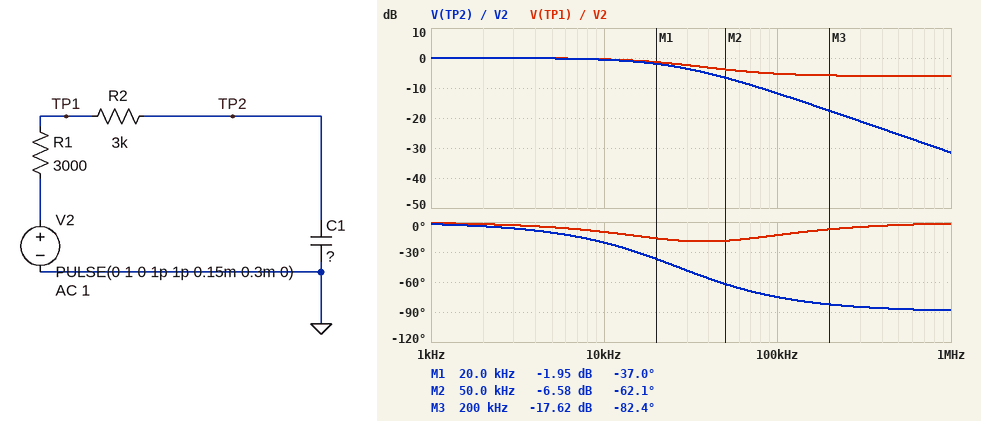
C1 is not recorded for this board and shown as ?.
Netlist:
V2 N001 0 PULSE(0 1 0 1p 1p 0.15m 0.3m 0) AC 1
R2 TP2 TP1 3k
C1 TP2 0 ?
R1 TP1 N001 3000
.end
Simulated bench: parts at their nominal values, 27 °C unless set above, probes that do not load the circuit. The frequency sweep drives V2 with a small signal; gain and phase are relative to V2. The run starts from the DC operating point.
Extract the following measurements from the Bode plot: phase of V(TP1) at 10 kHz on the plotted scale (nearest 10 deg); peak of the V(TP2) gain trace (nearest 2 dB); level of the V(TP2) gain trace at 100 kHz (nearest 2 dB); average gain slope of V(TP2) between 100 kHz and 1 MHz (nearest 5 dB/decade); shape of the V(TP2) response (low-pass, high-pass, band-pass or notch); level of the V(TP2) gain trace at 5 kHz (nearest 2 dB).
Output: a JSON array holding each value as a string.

["-10 deg", "0 dB", "-12 dB", "-20 dB/decade", "low-pass", "0 dB"]
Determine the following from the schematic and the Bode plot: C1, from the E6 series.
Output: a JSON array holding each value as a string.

["1 nF"]
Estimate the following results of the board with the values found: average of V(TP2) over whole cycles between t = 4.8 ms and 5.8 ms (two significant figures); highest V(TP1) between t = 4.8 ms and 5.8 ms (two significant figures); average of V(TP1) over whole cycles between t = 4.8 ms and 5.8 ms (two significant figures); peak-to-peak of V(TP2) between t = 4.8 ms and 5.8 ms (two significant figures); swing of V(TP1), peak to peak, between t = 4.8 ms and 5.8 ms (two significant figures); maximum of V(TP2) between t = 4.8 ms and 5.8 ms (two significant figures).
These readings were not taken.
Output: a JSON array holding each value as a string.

["500 mV", "1.0 V", "500 mV", "1.0 V", "1.0 V", "1.0 V"]
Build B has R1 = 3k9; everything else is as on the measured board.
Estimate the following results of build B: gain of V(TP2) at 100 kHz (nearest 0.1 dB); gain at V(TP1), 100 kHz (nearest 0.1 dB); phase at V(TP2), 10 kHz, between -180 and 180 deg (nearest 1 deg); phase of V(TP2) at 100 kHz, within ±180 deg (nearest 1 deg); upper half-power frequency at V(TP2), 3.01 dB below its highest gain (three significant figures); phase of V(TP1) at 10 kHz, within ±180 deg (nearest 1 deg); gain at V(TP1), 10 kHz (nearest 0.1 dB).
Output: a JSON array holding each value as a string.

["-13.0 dB", "-6.4 dB", "-23 deg", "-77 deg", "23.1 kHz", "-13 deg", "-0.6 dB"]
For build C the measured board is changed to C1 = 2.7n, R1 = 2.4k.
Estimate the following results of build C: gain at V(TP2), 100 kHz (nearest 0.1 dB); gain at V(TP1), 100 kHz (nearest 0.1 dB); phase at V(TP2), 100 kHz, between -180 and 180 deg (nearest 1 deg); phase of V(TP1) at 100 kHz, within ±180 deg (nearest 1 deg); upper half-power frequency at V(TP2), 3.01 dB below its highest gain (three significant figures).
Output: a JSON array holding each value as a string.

["-19.3 dB", "-5.0 dB", "-84 deg", "-5 deg", "10.9 kHz"]
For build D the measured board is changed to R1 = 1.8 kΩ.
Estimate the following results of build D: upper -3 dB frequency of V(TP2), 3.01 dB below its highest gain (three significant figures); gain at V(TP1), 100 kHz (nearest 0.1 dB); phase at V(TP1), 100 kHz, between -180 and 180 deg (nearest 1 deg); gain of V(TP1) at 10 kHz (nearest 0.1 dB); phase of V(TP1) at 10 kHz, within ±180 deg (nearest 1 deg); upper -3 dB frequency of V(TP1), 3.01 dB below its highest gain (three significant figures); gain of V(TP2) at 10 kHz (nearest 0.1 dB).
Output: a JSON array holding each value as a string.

["33.2 kHz", "-3.5 dB", "-10 deg", "-0.2 dB", "-6 deg", "70.9 kHz", "-0.4 dB"]
